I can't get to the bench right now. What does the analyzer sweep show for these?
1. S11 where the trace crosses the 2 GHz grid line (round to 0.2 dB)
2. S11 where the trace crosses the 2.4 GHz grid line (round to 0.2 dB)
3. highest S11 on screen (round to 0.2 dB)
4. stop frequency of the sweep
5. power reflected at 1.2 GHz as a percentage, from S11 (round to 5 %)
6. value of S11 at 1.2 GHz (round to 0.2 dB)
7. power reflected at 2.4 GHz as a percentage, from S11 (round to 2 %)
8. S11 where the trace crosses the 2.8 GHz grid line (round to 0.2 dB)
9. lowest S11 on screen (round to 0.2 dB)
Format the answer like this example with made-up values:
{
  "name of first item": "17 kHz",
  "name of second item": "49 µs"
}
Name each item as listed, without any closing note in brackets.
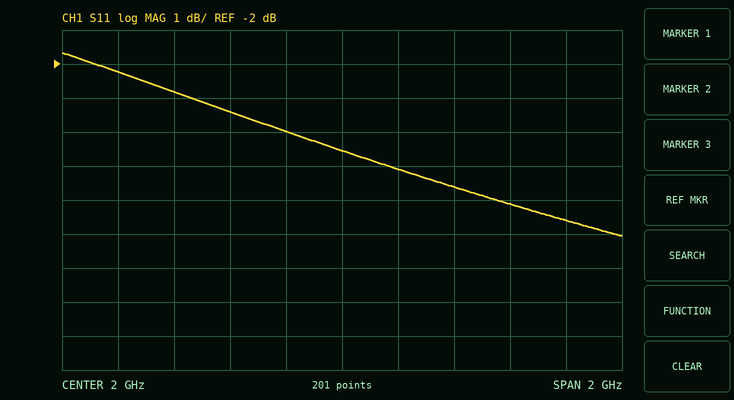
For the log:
{
  "S11 where the trace crosses the 2 GHz grid line": "-4.6 dB",
  "S11 where the trace crosses the 2.4 GHz grid line": "-5.6 dB",
  "highest S11 on screen": "-1.6 dB",
  "stop frequency of the sweep": "3 GHz",
  "power reflected at 1.2 GHz as a percentage, from S11": "60 %",
  "value of S11 at 1.2 GHz": "-2.2 dB",
  "power reflected at 2.4 GHz as a percentage, from S11": "28 %",
  "S11 where the trace crosses the 2.8 GHz grid line": "-6.6 dB",
  "lowest S11 on screen": "-7.0 dB"
}
